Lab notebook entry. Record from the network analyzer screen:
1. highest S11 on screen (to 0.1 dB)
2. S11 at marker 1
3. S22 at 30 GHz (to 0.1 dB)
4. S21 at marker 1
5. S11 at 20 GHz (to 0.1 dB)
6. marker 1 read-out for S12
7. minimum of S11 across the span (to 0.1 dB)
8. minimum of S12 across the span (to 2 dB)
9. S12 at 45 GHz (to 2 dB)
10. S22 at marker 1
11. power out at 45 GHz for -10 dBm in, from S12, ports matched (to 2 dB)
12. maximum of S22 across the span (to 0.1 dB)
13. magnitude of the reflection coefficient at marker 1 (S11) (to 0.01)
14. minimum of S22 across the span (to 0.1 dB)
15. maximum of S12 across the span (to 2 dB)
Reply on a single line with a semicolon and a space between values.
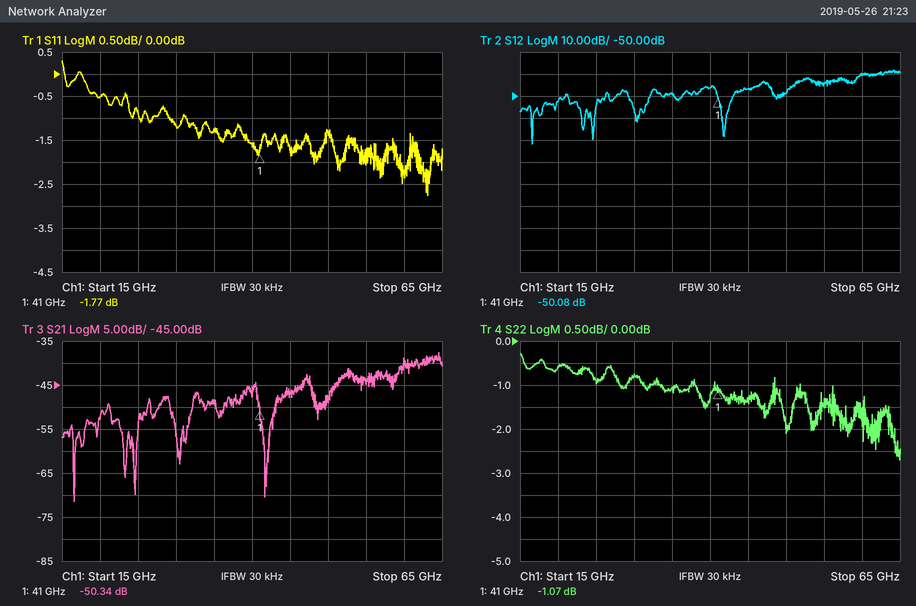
0.3 dB; -1.77 dB; -0.8 dB; -50.34 dB; -0.5 dB; -50.08 dB; -2.8 dB; -72 dB; -46 dB; -1.07 dB; -56 dBm; -0.3 dB; 0.82; -2.7 dB; -38 dB
